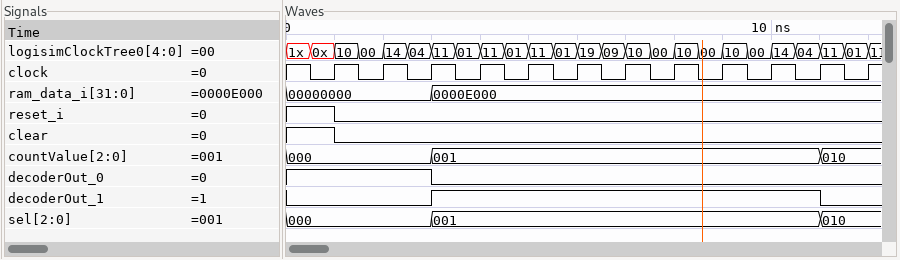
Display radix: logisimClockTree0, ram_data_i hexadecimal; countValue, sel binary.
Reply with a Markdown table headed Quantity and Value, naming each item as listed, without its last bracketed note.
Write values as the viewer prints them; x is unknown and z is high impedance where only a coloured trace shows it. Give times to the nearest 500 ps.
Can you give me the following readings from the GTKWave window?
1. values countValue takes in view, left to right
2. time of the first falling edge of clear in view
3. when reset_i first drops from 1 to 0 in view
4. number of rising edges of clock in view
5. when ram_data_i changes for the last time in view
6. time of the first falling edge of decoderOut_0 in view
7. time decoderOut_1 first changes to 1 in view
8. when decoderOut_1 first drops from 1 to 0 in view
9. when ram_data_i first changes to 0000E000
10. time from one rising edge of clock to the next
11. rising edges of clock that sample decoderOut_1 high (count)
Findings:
| Quantity | Value |
|---|---|
| values countValue takes in view, left to right | 000, 001, 010 |
| time of the first falling edge of clear in view | 1000 ps |
| when reset_i first drops from 1 to 0 in view | 1000 ps |
| number of rising edges of clock in view | 12 |
| when ram_data_i changes for the last time in view | 3000 ps |
| time of the first falling edge of decoderOut_0 in view | 3000 ps |
| time decoderOut_1 first changes to 1 in view | 3000 ps |
| when decoderOut_1 first drops from 1 to 0 in view | 11000 ps |
| when ram_data_i first changes to 0000E000 | 3000 ps |
| time from one rising edge of clock to the next | 1000 ps |
| rising edges of clock that sample decoderOut_1 high | 8 |
